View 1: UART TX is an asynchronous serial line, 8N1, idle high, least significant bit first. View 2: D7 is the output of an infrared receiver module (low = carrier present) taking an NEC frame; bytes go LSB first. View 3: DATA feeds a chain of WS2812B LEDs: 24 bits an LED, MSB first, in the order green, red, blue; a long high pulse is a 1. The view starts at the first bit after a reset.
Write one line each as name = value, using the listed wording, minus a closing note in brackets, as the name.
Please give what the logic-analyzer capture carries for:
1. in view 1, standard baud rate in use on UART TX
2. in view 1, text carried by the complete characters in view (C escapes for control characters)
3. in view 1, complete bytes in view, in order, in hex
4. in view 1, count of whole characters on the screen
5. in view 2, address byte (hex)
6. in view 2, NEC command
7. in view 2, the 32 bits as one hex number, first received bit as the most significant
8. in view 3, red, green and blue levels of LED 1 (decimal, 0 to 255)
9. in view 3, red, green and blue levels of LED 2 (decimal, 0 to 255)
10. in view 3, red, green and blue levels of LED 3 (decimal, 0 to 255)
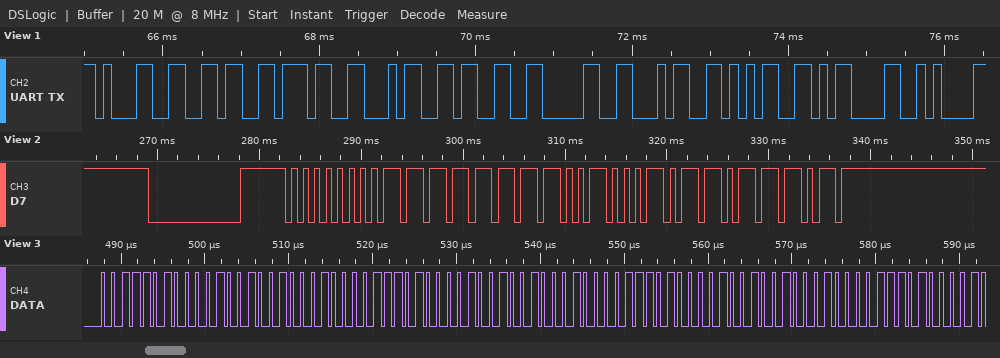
in view 1, standard baud rate in use on UART TX = 9600 baud
in view 1, text carried by the complete characters in view = "16743045\r\n"
in view 1, complete bytes in view, in order, in hex = 31 36 37 34 33 30 34 35 0D 0A
in view 1, count of whole characters on the screen = 10
in view 2, address byte = 0x00
in view 2, NEC command = 0x44
in view 2, the 32 bits as one hex number, first received bit as the most significant = 0x00FF22DD
in view 3, red, green and blue levels of LED 1 = 18, 58, 68
in view 3, red, green and blue levels of LED 2 = 18, 58, 68
in view 3, red, green and blue levels of LED 3 = 18, 58, 68
